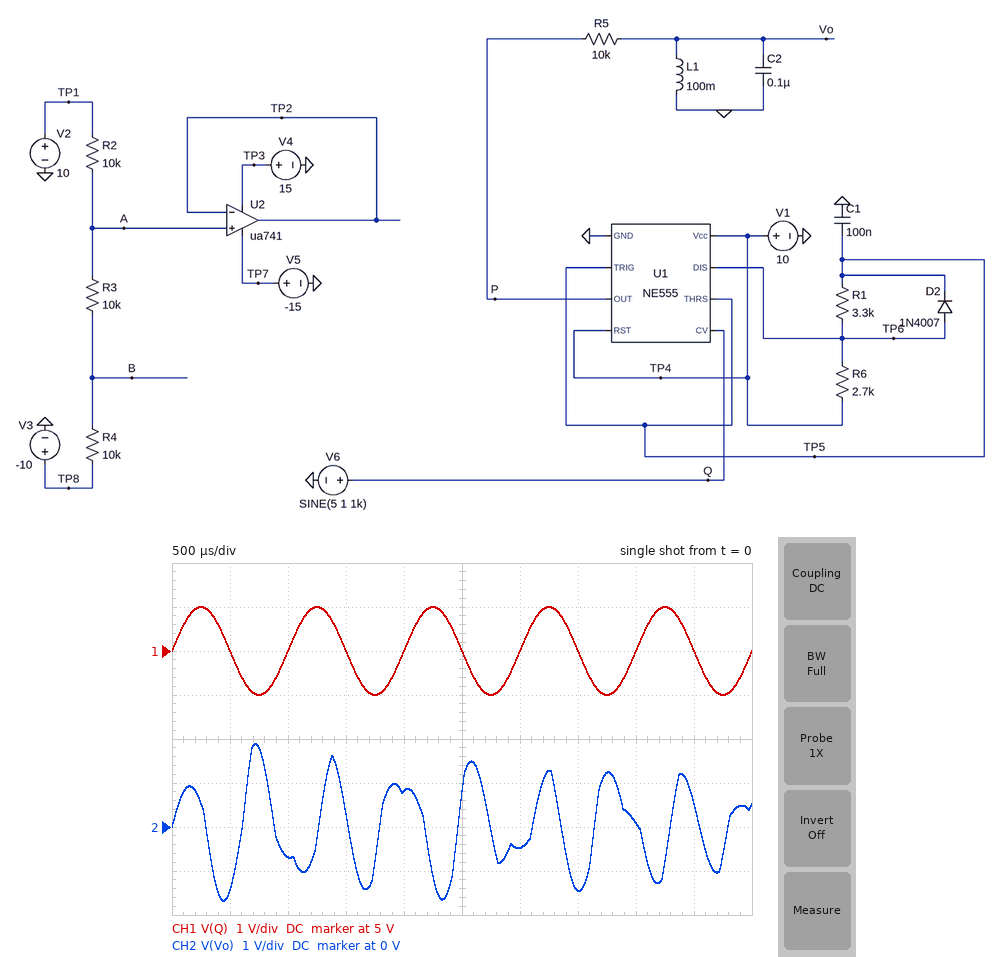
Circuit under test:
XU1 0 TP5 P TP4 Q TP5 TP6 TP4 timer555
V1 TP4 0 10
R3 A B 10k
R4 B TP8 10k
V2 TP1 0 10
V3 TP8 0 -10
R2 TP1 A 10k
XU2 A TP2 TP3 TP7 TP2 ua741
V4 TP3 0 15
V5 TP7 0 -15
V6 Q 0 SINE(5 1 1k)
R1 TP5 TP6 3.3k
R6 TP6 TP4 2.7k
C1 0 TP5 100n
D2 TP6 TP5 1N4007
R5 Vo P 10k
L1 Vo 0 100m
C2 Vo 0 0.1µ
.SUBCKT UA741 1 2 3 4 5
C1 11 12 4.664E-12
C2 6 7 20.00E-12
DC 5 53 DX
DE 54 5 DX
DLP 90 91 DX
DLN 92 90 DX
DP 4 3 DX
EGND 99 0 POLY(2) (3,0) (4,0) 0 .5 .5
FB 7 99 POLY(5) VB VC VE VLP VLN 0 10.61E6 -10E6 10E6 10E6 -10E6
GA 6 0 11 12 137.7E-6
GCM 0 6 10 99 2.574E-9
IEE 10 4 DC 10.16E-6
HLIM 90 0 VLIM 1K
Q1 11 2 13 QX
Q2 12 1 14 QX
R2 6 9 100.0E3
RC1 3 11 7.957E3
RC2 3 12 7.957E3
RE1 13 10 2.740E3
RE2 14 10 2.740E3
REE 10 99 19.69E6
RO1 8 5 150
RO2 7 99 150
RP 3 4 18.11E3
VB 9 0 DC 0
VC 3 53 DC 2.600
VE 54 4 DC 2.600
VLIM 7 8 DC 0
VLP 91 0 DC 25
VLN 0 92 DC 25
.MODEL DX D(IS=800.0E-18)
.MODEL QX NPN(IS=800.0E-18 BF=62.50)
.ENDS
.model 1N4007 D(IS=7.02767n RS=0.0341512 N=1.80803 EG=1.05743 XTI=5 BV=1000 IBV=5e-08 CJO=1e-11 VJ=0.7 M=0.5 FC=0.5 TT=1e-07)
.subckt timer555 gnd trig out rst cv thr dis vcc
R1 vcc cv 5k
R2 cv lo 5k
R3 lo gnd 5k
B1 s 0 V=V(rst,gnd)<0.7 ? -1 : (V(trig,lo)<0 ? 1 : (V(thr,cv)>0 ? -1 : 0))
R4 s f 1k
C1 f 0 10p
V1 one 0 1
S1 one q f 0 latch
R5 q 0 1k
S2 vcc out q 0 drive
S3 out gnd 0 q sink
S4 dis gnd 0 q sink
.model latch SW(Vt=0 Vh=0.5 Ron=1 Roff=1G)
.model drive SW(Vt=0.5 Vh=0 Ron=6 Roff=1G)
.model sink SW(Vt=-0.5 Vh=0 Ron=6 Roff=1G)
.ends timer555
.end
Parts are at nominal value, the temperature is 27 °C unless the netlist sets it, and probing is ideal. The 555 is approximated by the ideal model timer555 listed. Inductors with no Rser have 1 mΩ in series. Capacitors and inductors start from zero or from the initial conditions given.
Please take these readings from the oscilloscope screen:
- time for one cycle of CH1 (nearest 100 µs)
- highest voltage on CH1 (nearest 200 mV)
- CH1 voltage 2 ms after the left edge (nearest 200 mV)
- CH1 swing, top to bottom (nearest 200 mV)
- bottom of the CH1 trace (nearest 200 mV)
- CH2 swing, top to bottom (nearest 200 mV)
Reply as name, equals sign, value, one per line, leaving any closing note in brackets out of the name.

time for one cycle of CH1 = 1.0 ms
highest voltage on CH1 = 6.0 V
CH1 voltage 2 ms after the left edge = 5.0 V
CH1 swing, top to bottom = 2.0 V
bottom of the CH1 trace = 4.0 V
CH2 swing, top to bottom = 3.6 V
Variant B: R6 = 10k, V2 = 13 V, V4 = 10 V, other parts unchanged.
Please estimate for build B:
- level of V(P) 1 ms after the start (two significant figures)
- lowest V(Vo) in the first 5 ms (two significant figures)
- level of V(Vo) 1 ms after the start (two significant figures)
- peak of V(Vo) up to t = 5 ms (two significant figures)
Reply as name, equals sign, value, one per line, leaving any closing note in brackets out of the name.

level of V(P) 1 ms after the start = 10 V
lowest V(Vo) in the first 5 ms = -1.0 V
level of V(Vo) 1 ms after the start = 1.1 V
peak of V(Vo) up to t = 5 ms = 1.2 V
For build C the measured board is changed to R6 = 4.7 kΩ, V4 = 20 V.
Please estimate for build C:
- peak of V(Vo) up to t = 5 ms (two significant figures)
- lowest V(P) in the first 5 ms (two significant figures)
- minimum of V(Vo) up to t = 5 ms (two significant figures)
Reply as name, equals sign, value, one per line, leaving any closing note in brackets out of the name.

peak of V(Vo) up to t = 5 ms = 2.1 V
lowest V(P) in the first 5 ms = -1.6 mV
minimum of V(Vo) up to t = 5 ms = -2.6 V
